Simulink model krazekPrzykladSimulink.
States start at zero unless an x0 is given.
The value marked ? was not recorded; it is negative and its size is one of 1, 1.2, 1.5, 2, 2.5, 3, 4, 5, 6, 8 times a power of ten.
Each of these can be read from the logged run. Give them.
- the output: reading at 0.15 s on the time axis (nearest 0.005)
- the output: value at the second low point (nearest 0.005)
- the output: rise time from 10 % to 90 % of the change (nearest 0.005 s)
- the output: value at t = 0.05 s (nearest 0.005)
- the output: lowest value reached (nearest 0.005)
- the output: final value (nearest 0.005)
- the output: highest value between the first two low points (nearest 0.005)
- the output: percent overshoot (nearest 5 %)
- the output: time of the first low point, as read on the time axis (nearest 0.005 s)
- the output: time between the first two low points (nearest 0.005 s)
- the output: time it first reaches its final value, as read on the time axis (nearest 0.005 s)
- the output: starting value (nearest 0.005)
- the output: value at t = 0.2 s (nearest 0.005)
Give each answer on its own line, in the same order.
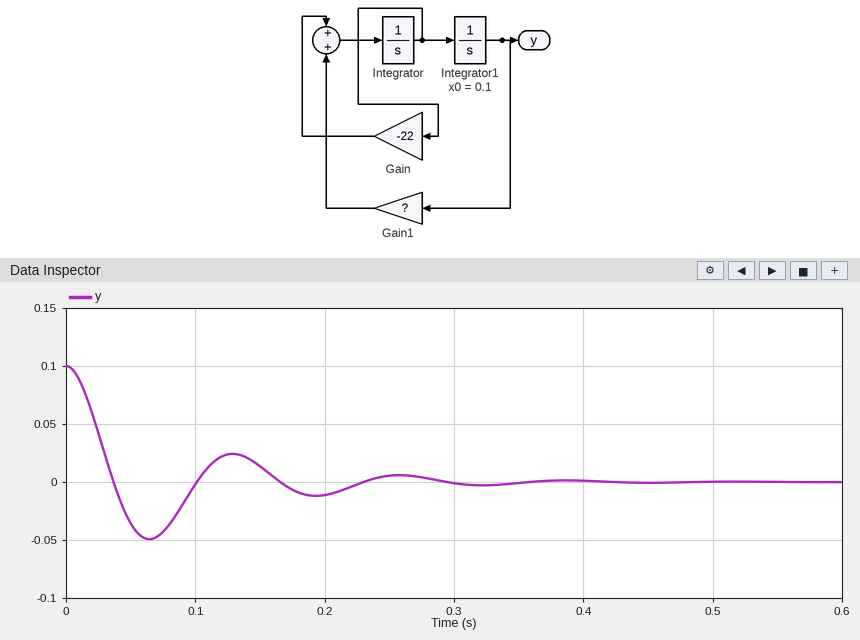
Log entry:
0.015
-0.010
0.025 s
-0.035
-0.050
0.000
0.025
50 %
0.065 s
0.130 s
0.035 s
0.100
-0.010
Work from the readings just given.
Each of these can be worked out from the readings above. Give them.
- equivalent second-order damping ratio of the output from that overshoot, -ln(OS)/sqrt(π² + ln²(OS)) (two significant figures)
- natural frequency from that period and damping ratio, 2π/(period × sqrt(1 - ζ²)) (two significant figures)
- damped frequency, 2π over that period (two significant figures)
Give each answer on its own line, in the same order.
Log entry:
0.22
50 rad/s
48 rad/s
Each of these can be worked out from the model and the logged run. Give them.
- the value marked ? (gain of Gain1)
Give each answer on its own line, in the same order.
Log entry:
-2500
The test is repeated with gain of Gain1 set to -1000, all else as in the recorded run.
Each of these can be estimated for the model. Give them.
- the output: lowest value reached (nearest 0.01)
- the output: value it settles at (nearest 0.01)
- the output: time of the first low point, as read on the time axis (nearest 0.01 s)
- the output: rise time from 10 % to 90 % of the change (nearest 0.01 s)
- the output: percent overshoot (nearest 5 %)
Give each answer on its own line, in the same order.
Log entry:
-0.03
0.00
0.11 s
0.04 s
30 %
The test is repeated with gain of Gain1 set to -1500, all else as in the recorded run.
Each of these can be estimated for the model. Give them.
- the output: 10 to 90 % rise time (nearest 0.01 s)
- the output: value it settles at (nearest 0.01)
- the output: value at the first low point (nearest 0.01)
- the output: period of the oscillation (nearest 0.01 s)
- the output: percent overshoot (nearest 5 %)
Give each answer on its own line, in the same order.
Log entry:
0.03 s
0.00
-0.04
0.17 s
40 %
